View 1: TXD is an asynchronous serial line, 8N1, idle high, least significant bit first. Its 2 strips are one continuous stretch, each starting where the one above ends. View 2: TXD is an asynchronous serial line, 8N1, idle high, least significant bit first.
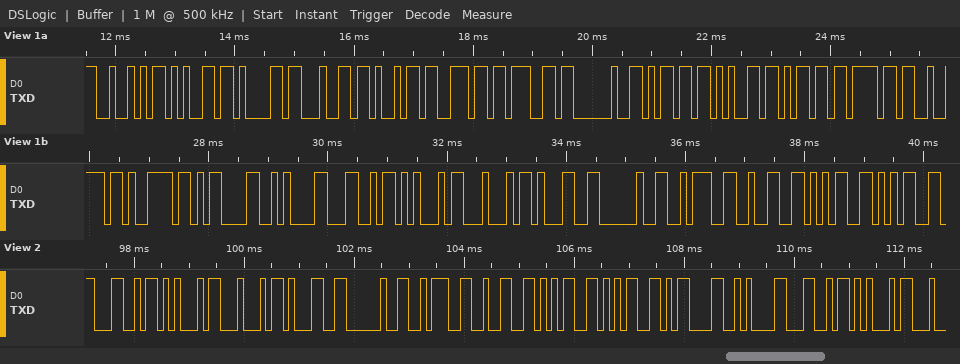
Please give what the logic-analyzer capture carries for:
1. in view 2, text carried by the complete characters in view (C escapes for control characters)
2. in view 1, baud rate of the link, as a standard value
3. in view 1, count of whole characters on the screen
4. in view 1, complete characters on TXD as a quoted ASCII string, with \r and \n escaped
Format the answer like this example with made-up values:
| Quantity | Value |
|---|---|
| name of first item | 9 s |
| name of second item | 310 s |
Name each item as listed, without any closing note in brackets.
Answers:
| Quantity | Value |
|---|---|
| in view 2, text carried by the complete characters in view | "LED1 :255\r\nLE" |
| in view 1, baud rate of the link, as a standard value | 9600 baud |
| in view 1, count of whole characters on the screen | 25 |
| in view 1, complete characters on TXD as a quoted ASCII string, with \r and \n escaped | "Reading memory\r\nLED1 :255" |
